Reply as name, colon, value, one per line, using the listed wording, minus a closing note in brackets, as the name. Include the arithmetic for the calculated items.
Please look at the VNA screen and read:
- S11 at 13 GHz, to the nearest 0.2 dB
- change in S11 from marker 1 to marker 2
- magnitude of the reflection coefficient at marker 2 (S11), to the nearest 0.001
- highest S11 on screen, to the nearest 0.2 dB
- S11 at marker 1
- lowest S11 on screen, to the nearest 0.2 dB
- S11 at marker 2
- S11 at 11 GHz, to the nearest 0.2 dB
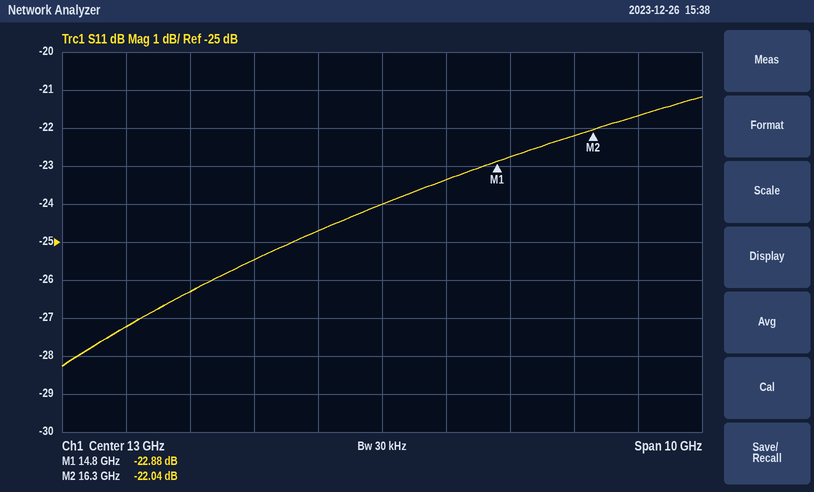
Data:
S11 at 13 GHz, to the nearest 0.2 dB: -24.0 dB
change in S11 from marker 1 to marker 2: -22.04 − (-22.88) = 0.84 dB
magnitude of the reflection coefficient at marker 2 (S11), to the nearest 0.001: 10^(-22.04/20) ≈ 0.079
highest S11 on screen, to the nearest 0.2 dB: -21.2 dB
S11 at marker 1: -22.88 dB
lowest S11 on screen, to the nearest 0.2 dB: -28.2 dB
S11 at marker 2: -22.04 dB
S11 at 11 GHz, to the nearest 0.2 dB: -25.4 dB
